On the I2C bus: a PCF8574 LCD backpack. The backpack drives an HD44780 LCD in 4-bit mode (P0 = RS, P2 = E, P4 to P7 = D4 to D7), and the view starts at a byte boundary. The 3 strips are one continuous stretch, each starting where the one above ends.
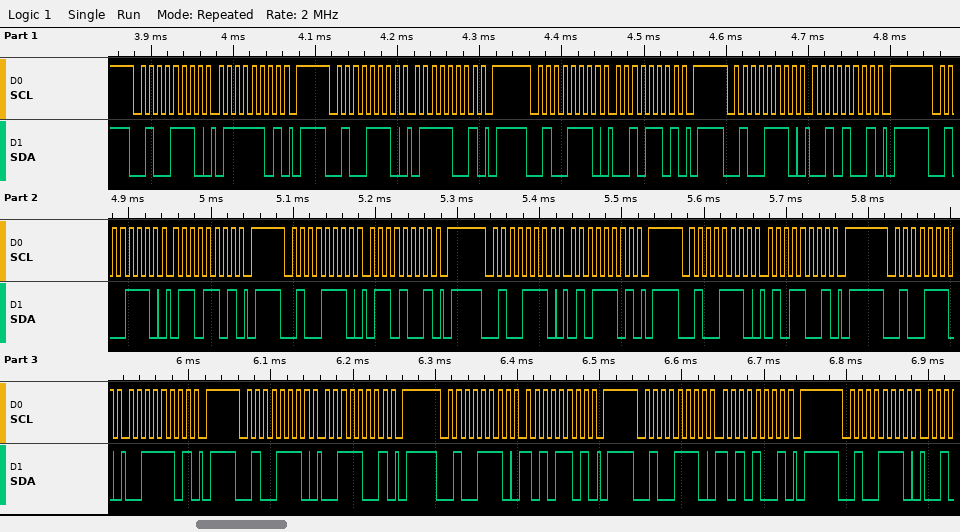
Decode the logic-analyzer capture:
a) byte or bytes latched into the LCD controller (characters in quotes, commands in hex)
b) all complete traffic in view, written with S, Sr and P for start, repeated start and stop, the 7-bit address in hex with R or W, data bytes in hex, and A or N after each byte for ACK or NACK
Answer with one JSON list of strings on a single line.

["'r' 'e' ':'", "S 27W A 7D A P S 27W A 79 A P S 27W A 2D A P S 27W A 29 A P S 27W A 6D A P S 27W A 69 A P S 27W A 5D A P S 27W A 59 A P S 27W A 3D A P S 27W A 39 A P S 27W A AD A P S 27W A A9 A P S 27W A"]
